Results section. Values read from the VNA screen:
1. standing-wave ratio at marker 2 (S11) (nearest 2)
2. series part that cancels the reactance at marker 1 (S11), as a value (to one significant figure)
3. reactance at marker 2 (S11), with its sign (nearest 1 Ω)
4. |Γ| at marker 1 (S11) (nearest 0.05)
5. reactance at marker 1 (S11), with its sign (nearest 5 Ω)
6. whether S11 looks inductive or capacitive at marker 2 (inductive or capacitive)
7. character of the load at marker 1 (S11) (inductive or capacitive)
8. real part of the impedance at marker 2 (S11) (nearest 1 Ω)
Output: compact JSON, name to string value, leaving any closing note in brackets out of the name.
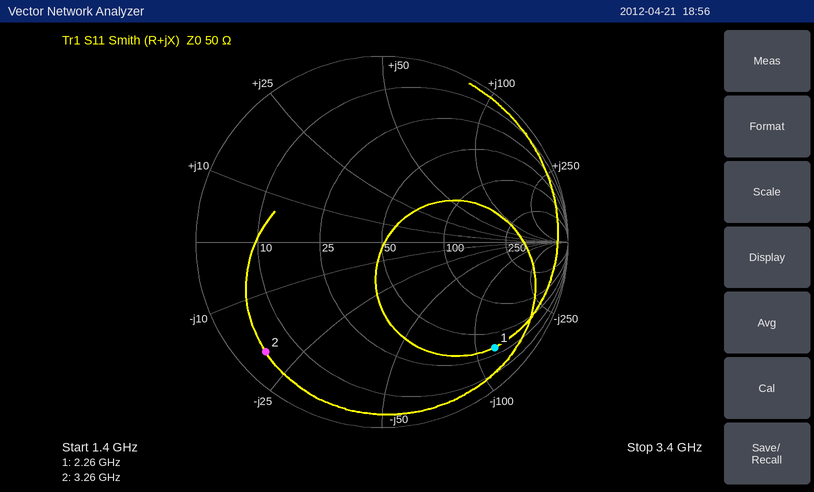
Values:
{"standing-wave ratio at marker 2 (S11)": "14", "series part that cancels the reactance at marker 1 (S11), as a value": "8 nH", "reactance at marker 2 (S11), with its sign": "-20 Ω", "|Γ| at marker 1 (S11)": "0.85", "reactance at marker 1 (S11), with its sign": "-120 Ω", "whether S11 looks inductive or capacitive at marker 2": "capacitive", "character of the load at marker 1 (S11)": "capacitive", "real part of the impedance at marker 2 (S11)": "4 Ω"}
